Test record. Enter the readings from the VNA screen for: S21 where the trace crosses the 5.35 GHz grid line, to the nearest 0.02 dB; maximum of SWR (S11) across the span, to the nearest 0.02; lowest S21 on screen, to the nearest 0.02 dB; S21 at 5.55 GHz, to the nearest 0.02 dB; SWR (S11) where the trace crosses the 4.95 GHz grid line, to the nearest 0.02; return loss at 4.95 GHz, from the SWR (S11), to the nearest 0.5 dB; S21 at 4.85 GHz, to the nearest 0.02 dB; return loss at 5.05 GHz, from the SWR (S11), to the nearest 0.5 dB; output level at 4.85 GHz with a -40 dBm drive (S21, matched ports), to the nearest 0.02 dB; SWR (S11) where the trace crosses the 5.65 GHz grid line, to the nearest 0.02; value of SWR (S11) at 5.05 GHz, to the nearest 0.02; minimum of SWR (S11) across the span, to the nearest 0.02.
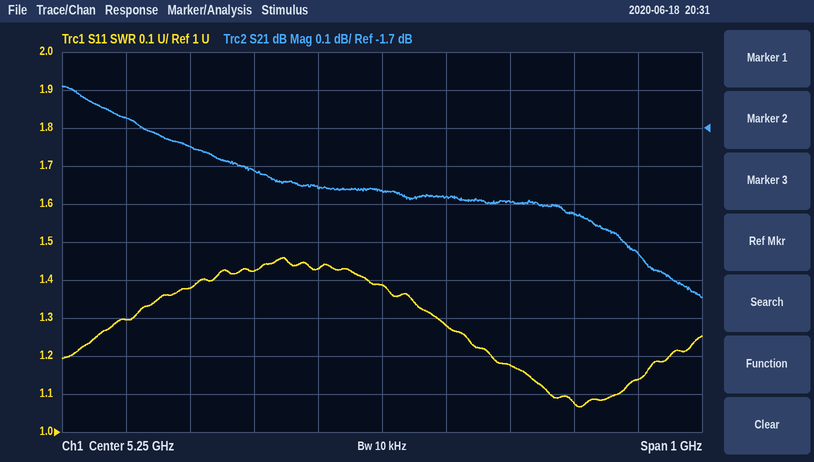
-1.88 dB
1.46
-2.14 dB
-1.92 dB
1.38
16.0 dB
-1.68 dB
15.0 dB
-41.68 dBm
1.14
1.42
1.06
